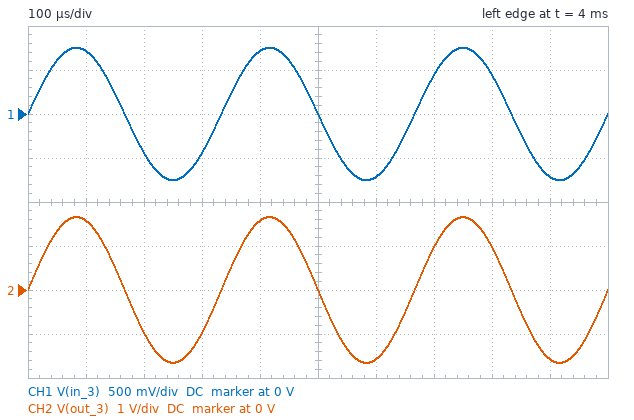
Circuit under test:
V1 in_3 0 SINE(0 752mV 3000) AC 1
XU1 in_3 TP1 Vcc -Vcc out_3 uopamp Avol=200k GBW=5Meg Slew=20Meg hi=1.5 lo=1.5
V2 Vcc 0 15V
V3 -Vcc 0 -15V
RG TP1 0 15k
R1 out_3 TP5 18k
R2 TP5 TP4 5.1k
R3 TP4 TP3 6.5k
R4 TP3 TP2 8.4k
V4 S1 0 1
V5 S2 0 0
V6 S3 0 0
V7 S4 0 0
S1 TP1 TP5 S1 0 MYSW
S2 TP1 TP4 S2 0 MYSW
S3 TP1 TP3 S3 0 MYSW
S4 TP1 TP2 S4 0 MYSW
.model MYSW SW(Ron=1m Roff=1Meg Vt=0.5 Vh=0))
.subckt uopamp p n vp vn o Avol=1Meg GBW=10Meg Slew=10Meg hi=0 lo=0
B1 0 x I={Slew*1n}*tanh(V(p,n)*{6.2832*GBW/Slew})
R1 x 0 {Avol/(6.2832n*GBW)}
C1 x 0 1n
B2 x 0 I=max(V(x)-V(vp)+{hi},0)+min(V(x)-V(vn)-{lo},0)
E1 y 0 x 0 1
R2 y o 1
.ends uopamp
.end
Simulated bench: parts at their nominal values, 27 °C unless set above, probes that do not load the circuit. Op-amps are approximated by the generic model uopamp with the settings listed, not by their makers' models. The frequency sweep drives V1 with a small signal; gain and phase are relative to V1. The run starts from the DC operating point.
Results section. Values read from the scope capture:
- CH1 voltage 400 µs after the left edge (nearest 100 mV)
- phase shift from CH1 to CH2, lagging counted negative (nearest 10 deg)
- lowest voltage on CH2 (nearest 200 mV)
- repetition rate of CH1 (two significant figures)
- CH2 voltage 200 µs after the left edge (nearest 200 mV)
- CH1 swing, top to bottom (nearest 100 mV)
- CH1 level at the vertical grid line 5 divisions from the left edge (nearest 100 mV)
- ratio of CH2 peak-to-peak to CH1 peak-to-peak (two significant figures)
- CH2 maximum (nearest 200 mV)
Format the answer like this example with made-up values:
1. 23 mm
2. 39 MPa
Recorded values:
1. 700 mV
2. 0 deg
3. -1.6 V
4. 3.0 kHz
5. -1.0 V
6. 1.5 V
7. 0 V
8. 2.2
9. 1.6 V
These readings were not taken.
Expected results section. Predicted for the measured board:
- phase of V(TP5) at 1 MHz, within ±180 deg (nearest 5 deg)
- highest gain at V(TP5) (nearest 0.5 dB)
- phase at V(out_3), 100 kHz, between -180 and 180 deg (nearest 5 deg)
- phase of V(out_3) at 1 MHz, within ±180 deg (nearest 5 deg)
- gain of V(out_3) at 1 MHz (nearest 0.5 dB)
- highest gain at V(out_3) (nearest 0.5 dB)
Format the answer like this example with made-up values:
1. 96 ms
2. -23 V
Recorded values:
1. -75 deg
2. 25.0 dB
3. -20 deg
4. -75 deg
5. 13.5 dB
6. 25.5 dB
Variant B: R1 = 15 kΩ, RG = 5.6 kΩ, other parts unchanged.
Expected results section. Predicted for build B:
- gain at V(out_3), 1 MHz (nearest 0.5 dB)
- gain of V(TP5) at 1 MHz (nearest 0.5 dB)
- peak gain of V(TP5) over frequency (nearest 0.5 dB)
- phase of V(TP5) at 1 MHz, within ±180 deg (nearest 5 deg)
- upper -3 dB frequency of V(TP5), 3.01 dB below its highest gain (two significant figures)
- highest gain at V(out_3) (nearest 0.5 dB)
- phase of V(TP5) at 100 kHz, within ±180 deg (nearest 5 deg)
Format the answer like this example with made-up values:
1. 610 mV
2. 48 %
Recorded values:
1. 14.0 dB
2. 13.5 dB
3. 33.5 dB
4. -85 deg
5. 100 kHz
6. 34.0 dB
7. -45 deg
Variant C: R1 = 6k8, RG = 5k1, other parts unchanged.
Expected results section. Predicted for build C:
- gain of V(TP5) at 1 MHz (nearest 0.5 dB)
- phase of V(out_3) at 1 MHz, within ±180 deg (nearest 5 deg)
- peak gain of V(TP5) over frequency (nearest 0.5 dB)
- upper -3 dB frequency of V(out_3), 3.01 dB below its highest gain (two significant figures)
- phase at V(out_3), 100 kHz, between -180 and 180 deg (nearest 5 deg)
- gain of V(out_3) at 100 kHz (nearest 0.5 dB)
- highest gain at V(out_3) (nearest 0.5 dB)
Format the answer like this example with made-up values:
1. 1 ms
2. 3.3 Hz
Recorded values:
1. 13.5 dB
2. -85 deg
3. 34.0 dB
4. 96 kHz
5. -45 deg
6. 31.0 dB
7. 34.5 dB
